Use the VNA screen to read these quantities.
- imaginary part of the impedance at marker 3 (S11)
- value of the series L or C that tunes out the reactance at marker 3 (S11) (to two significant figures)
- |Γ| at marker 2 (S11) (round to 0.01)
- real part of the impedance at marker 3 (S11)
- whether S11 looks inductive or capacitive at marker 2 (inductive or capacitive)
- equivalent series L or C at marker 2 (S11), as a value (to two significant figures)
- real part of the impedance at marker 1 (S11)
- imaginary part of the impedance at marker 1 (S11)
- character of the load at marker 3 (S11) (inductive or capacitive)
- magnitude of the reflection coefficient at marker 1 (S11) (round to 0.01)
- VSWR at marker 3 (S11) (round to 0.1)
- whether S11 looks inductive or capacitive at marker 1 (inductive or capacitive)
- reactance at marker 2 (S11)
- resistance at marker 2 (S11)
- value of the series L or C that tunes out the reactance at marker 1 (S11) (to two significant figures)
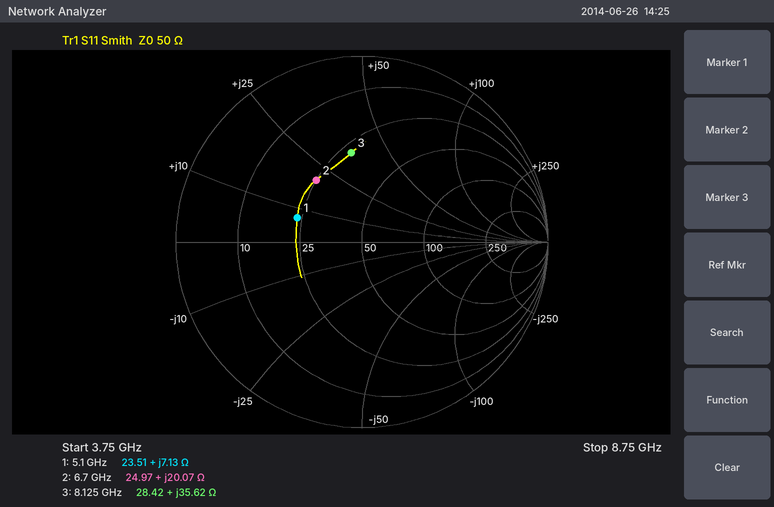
+35.62 Ω
550 fF
0.41
28.42 Ω
inductive
480 pH
23.51 Ω
+7.13 Ω
inductive
0.37
2.9
inductive
+20.07 Ω
24.97 Ω
4.4 pF
